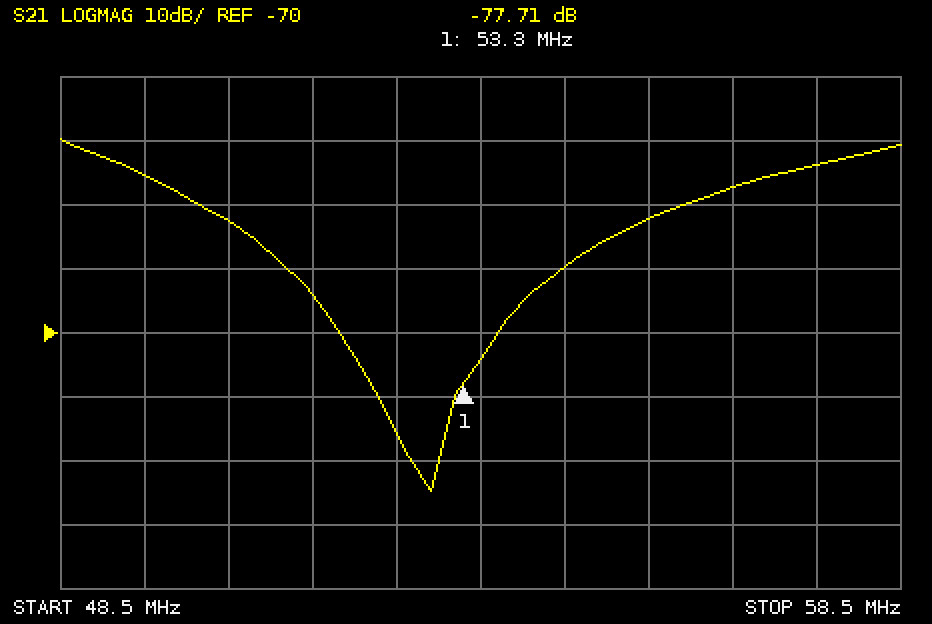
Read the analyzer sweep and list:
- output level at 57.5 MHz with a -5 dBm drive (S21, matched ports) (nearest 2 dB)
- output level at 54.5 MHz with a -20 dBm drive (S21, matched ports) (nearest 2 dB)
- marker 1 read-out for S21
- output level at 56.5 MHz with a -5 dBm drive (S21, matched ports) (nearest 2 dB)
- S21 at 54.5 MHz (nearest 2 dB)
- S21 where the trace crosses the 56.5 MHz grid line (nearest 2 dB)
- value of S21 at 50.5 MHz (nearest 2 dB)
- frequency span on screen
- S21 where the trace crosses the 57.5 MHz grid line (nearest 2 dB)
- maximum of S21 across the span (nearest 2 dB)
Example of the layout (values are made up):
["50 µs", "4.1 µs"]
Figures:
["-48 dBm", "-80 dBm", "-77.71 dB", "-52 dBm", "-60 dB", "-48 dB", "-52 dB", "10 MHz", "-44 dB", "-40 dB"]
